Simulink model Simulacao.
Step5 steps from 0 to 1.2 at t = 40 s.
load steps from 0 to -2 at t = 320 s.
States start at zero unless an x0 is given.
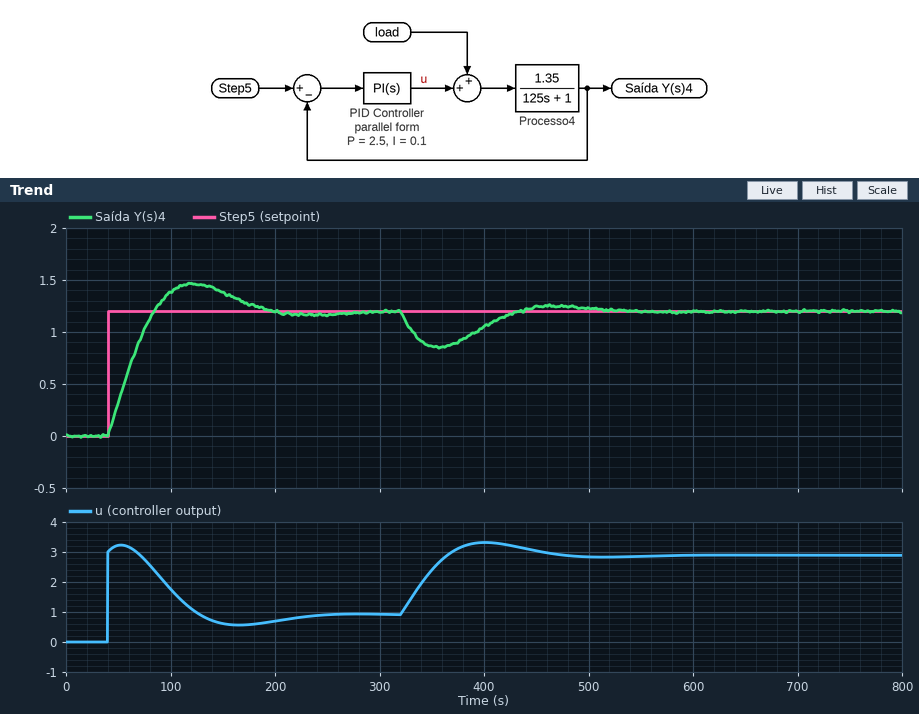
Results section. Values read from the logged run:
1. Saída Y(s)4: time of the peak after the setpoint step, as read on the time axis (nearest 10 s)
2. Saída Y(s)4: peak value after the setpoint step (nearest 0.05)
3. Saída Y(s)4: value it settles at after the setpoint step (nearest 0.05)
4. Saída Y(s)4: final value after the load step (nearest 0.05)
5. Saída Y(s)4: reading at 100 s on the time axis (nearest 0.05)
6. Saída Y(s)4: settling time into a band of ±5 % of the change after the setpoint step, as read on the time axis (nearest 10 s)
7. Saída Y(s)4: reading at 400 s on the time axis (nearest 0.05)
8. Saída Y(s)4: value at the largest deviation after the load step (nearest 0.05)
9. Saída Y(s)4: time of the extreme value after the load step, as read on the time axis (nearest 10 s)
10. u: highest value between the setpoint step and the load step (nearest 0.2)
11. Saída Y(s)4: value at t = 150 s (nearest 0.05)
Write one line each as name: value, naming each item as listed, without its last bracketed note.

Saída Y(s)4: time of the peak after the setpoint step, as read on the time axis: 120 s
Saída Y(s)4: peak value after the setpoint step: 1.45
Saída Y(s)4: value it settles at after the setpoint step: 1.20
Saída Y(s)4: final value after the load step: 1.20
Saída Y(s)4: reading at 100 s on the time axis: 1.40
Saída Y(s)4: settling time into a band of ±5 % of the change after the setpoint step, as read on the time axis: 180 s
Saída Y(s)4: reading at 400 s on the time axis: 1.05
Saída Y(s)4: value at the largest deviation after the load step: 0.85
Saída Y(s)4: time of the extreme value after the load step, as read on the time axis: 360 s
u: highest value between the setpoint step and the load step: 3.2
Saída Y(s)4: value at t = 150 s: 1.40
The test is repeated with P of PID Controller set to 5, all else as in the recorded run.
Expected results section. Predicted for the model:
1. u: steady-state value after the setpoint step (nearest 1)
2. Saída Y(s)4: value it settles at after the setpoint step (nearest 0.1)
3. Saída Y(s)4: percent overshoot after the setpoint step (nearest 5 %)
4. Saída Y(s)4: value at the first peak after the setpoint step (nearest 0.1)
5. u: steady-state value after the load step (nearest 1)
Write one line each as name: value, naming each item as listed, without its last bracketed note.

u: steady-state value after the setpoint step: 1
Saída Y(s)4: value it settles at after the setpoint step: 1.2
Saída Y(s)4: percent overshoot after the setpoint step: 10 %
Saída Y(s)4: value at the first peak after the setpoint step: 1.3
u: steady-state value after the load step: 3
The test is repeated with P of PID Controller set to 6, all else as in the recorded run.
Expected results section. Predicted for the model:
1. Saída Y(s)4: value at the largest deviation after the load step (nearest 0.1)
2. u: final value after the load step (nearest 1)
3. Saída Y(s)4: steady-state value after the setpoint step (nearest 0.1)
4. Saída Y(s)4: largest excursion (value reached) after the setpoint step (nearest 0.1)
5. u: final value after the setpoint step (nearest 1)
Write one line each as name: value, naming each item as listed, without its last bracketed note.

Saída Y(s)4: value at the largest deviation after the load step: 1.0
u: final value after the load step: 3
Saída Y(s)4: steady-state value after the setpoint step: 1.2
Saída Y(s)4: largest excursion (value reached) after the setpoint step: 1.3
u: final value after the setpoint step: 1
